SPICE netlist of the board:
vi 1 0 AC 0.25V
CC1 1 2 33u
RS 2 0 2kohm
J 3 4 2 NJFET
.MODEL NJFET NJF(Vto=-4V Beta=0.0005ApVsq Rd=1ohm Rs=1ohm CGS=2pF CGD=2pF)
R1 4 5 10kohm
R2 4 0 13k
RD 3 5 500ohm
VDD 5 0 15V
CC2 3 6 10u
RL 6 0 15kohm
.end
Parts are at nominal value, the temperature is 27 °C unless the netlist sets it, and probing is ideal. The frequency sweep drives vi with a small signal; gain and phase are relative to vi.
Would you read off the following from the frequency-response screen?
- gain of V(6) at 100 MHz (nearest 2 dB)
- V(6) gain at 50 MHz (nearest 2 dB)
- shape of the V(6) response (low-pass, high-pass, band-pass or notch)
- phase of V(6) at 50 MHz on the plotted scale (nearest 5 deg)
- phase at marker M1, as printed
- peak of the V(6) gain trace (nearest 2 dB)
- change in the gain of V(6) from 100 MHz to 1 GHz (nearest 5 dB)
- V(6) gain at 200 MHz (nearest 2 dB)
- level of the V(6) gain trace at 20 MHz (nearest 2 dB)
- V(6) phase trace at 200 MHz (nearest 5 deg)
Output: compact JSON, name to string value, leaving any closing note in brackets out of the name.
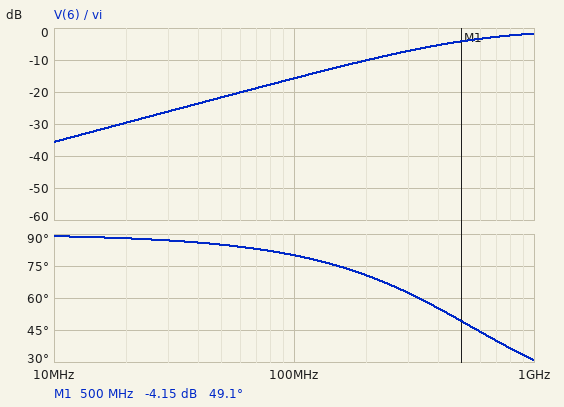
{"gain of V(6) at 100 MHz": "-16 dB", "V(6) gain at 50 MHz": "-22 dB", "shape of the V(6) response": "high-pass", "phase of V(6) at 50 MHz on the plotted scale": "85 deg", "phase at marker M1, as printed": "49.1 deg", "peak of the V(6) gain trace": "-2 dB", "change in the gain of V(6) from 100 MHz to 1 GHz": "15 dB", "V(6) gain at 200 MHz": "-10 dB", "level of the V(6) gain trace at 20 MHz": "-30 dB", "V(6) phase trace at 200 MHz": "70 deg"}
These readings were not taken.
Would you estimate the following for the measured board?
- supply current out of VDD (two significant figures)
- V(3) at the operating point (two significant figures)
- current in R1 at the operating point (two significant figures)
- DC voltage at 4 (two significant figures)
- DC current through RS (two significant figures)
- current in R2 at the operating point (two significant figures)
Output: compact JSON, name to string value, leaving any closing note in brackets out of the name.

{"supply current out of VDD": "1.2 mA", "V(3) at the operating point": "15 V", "current in R1 at the operating point": "1.2 mA", "DC voltage at 4": "2.7 V", "DC current through RS": "1.0 mA", "current in R2 at the operating point": "210 µA"}
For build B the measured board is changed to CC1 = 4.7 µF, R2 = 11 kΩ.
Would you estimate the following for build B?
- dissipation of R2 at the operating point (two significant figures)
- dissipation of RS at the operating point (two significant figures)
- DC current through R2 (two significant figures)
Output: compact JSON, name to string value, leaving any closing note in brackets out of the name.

{"dissipation of R2 at the operating point": "640 µW", "dissipation of RS at the operating point": "2.0 mW", "DC current through R2": "240 µA"}
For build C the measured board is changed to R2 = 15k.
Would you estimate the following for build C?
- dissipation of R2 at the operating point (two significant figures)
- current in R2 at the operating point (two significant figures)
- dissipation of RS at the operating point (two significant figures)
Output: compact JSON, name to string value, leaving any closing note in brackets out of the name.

{"dissipation of R2 at the operating point": "500 µW", "current in R2 at the operating point": "180 µA", "dissipation of RS at the operating point": "2.2 mW"}
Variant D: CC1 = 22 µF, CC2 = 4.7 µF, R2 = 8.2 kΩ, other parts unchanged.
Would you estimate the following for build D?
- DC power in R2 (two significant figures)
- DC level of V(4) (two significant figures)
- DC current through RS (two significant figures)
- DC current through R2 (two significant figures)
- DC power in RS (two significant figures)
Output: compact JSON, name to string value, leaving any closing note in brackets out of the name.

{"DC power in R2": "780 µW", "DC level of V(4)": "2.5 V", "DC current through RS": "940 µA", "DC current through R2": "310 µA", "DC power in RS": "1.8 mW"}
